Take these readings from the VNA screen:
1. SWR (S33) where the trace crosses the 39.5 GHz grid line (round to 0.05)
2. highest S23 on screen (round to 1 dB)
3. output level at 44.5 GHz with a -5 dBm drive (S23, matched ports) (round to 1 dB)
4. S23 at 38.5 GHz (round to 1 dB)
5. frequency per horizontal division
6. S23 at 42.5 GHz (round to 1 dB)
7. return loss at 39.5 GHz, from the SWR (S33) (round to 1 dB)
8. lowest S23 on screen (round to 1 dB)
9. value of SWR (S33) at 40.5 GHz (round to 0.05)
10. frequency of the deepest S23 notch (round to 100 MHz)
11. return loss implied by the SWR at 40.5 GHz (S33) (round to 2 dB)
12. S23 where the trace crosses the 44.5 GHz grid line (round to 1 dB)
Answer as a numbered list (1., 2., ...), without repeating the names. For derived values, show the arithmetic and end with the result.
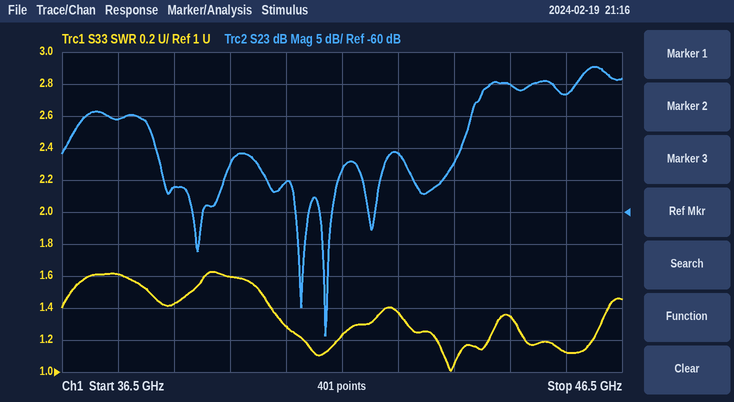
1. 1.60
2. -37 dB
3. -5 dBm + (-40 dB) = -45 dBm
4. -56 dB
5. 1 GHz
6. -51 dB
7. −20 log10((1.6 − 1)/(1.6 + 1)) ≈ 13 dB
8. -79 dB
9. 1.30
10. 41.2 GHz
11. −20 log10((1.3 − 1)/(1.3 + 1)) ≈ 18 dB
12. -40 dB
